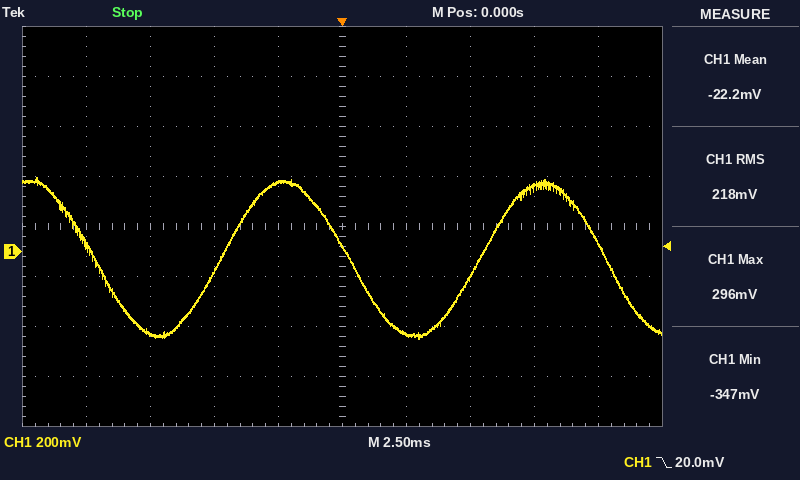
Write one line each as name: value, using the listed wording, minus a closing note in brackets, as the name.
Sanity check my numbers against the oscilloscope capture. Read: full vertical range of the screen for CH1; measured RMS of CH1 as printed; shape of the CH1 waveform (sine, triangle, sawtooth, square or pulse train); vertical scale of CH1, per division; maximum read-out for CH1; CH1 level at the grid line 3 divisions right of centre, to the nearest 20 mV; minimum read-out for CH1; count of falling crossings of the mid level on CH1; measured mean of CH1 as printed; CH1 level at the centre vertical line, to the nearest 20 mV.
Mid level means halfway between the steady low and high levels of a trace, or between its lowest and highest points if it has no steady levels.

full vertical range of the screen for CH1: 1.6 V
measured RMS of CH1 as printed: 218 mV
shape of the CH1 waveform: sine
vertical scale of CH1, per division: 200 mV
maximum read-out for CH1: 296 mV
CH1 level at the grid line 3 divisions right of centre, to the nearest 20 mV: 260 mV
minimum read-out for CH1: -347 mV
count of falling crossings of the mid level on CH1: 3
measured mean of CH1 as printed: -22.2 mV
CH1 level at the centre vertical line, to the nearest 20 mV: 20 mV
